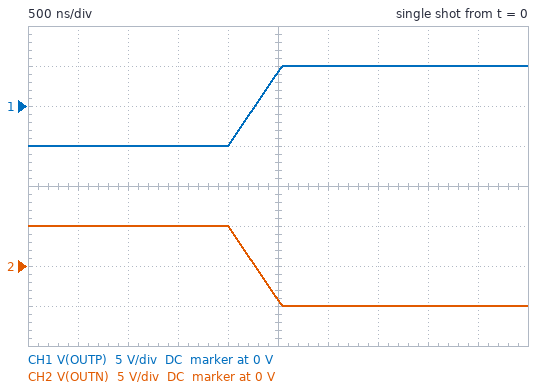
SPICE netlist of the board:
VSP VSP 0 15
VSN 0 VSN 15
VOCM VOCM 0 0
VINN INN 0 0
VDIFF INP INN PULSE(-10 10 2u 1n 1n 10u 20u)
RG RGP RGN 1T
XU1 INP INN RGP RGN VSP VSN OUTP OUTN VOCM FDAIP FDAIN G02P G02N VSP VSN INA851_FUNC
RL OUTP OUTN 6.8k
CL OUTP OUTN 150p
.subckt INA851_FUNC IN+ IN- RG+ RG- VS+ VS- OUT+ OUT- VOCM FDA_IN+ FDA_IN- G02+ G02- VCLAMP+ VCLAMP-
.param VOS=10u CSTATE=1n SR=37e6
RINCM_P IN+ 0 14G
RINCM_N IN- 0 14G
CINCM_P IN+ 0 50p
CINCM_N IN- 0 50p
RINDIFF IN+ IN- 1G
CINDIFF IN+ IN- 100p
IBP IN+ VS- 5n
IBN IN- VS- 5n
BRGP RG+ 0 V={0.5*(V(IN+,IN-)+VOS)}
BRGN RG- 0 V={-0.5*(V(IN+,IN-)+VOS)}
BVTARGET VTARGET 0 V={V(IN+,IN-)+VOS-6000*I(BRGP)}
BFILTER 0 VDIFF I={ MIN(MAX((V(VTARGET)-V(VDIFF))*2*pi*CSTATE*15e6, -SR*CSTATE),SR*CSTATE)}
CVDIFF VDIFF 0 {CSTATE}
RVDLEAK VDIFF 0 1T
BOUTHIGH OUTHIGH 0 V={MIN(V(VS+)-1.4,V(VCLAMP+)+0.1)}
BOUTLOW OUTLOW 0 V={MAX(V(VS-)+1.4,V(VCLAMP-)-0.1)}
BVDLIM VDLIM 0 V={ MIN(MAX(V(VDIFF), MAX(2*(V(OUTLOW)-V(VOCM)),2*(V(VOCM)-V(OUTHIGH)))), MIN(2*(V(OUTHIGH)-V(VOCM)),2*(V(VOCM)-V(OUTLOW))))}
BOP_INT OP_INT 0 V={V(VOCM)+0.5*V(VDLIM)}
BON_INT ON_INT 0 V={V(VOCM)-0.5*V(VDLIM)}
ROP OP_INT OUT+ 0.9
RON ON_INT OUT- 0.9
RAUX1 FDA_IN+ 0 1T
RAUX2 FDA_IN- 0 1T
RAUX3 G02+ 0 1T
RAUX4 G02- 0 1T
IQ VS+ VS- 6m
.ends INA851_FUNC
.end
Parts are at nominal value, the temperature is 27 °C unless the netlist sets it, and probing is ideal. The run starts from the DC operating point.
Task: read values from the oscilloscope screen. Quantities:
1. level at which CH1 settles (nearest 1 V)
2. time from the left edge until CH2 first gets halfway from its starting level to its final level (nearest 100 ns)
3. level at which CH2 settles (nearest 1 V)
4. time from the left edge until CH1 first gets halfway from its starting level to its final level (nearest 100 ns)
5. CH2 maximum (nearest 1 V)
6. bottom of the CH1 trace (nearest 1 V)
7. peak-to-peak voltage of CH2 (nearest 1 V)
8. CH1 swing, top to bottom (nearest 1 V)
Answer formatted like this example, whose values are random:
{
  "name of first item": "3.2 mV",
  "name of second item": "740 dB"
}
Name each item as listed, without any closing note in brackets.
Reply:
{
  "level at which CH1 settles": "5 V",
  "time from the left edge until CH2 first gets halfway from its starting level to its final level": "2.3 µs",
  "level at which CH2 settles": "-5 V",
  "time from the left edge until CH1 first gets halfway from its starting level to its final level": "2.3 µs",
  "CH2 maximum": "5 V",
  "bottom of the CH1 trace": "-5 V",
  "peak-to-peak voltage of CH2": "10 V",
  "CH1 swing, top to bottom": "10 V"
}
